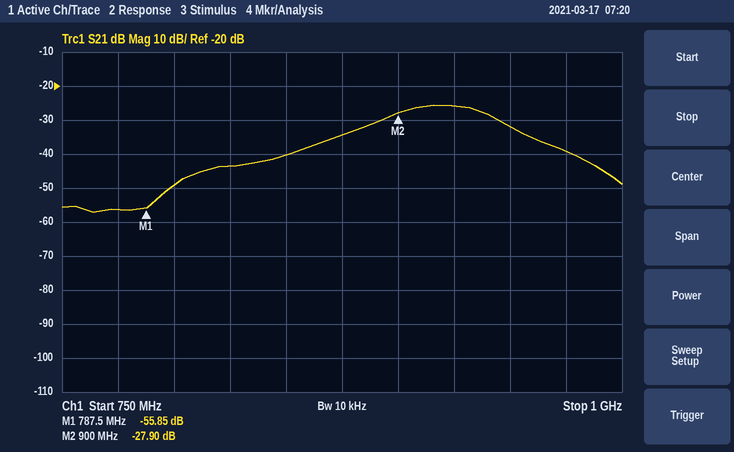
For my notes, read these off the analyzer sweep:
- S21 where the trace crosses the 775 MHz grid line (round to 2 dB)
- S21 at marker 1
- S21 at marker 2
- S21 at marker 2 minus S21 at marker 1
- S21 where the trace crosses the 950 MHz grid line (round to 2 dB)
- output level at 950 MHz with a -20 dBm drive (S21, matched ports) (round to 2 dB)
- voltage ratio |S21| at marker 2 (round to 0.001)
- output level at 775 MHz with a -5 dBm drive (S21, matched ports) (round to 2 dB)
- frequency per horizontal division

-56 dB
-55.85 dB
-27.90 dB
27.95 dB
-32 dB
-52 dBm
0.040
-62 dBm
25 MHz
